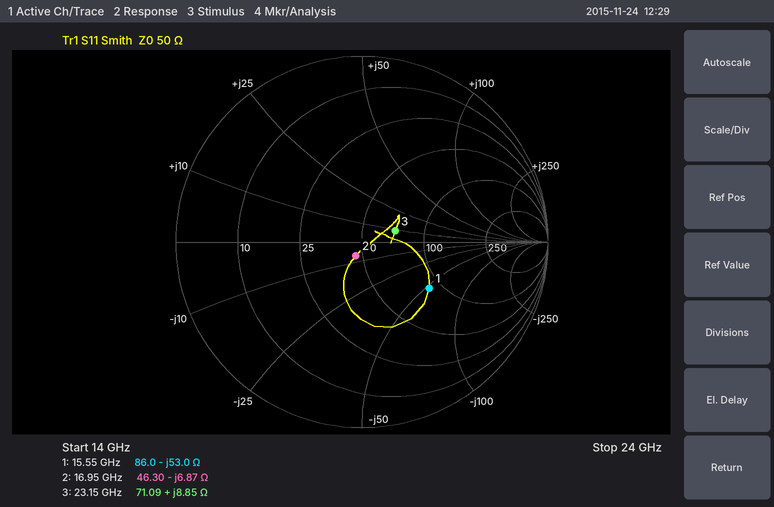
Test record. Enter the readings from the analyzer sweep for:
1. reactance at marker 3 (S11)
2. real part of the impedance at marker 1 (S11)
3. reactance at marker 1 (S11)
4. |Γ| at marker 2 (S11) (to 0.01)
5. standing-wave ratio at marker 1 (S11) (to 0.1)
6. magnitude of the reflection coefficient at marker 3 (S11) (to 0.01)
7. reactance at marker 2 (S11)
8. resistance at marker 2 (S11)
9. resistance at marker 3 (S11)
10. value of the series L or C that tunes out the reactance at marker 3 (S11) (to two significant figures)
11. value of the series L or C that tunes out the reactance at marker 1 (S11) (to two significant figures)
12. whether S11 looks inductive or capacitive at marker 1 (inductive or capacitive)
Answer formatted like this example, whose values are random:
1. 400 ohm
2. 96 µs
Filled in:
1. +8.85 Ω
2. 86.0 Ω
3. -53.0 Ω
4. 0.08
5. 2.6
6. 0.19
7. -6.87 Ω
8. 46.30 Ω
9. 71.09 Ω
10. 780 fF
11. 540 pH
12. capacitive
